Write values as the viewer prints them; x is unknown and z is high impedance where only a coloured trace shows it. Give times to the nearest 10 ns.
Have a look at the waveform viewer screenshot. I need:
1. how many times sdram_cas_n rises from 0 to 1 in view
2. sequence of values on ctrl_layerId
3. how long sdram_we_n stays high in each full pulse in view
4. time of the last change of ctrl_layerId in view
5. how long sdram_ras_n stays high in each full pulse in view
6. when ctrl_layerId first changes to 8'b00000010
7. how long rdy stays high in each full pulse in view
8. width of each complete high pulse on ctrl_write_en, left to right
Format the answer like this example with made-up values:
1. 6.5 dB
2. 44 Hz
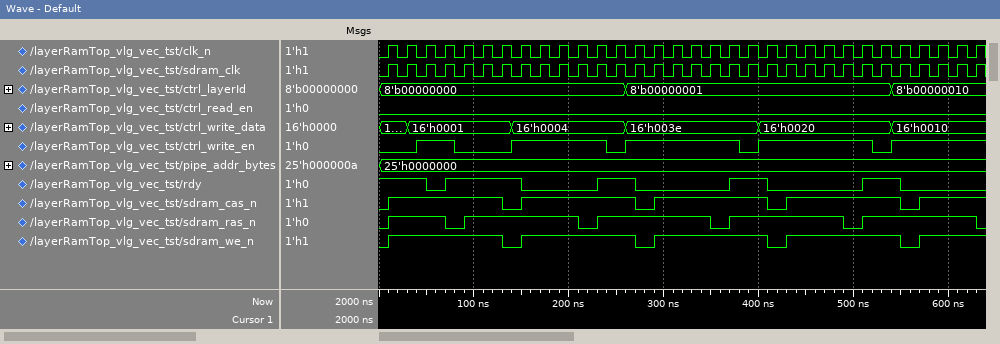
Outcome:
1. 5
2. 8'b00000000, 8'b00000001, 8'b00000010
3. 120 ns, 120 ns, 120 ns, 120 ns
4. 540 ns
5. 60 ns, 120 ns, 120 ns, 120 ns, 120 ns
6. 540 ns
7. 80 ns, 40 ns, 40 ns, 40 ns
8. 40 ns, 100 ns, 120 ns, 120 ns
